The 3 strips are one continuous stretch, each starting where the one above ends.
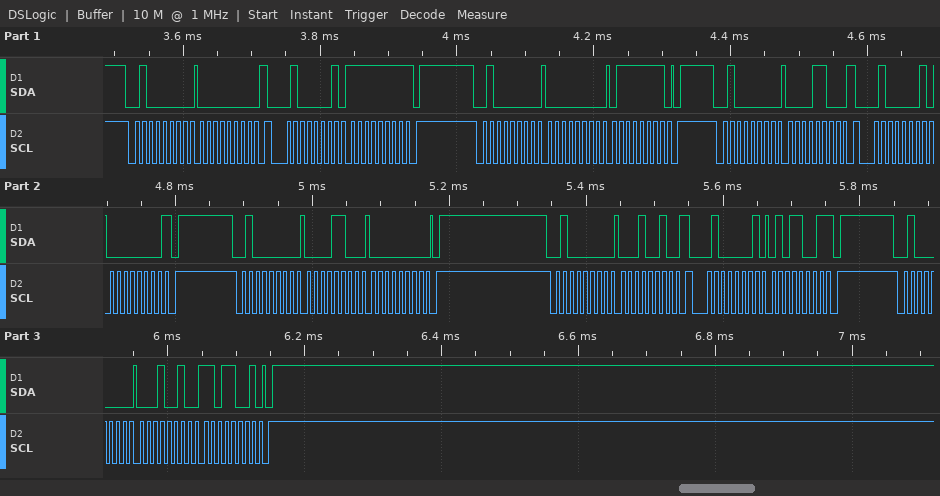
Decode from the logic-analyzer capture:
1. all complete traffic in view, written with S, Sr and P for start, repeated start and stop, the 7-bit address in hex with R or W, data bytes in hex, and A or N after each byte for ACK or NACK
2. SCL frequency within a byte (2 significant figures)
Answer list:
S 20W A 00 A Sr 20R A FF N P S 20W A 00 A 7F A P S 20W A 0C A Sr 20R A 00 N P S 20W A 0C A 00 A P S 20W A 12 A Sr 20R A 59 N P S 20W A 12 A D9 A P
100 kHz
